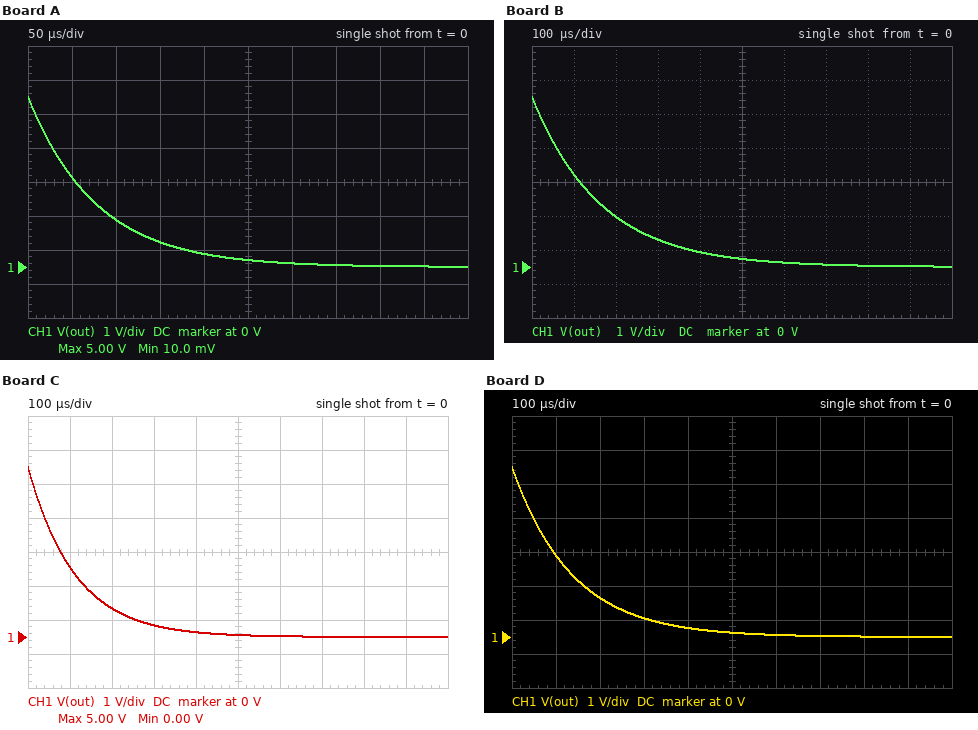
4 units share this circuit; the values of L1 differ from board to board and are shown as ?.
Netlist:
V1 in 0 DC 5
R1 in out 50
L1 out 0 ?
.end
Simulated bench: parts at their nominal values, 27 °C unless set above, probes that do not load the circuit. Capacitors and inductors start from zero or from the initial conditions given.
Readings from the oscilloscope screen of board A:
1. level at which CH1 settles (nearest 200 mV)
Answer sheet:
0 V
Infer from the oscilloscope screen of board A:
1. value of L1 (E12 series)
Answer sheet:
3.9 mH
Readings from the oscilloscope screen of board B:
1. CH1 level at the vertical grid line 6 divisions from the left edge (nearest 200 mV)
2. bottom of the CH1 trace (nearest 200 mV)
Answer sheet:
200 mV
0 V
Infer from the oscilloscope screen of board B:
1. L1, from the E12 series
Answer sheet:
8.2 mH
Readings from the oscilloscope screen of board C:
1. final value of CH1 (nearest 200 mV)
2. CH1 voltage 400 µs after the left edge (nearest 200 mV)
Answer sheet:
0 V
200 mV
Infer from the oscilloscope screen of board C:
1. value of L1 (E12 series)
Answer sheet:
5.6 mH
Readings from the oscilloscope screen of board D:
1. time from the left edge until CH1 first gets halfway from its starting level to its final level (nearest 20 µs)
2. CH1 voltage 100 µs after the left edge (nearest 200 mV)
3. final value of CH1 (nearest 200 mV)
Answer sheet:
100 µs
2.4 V
0 V
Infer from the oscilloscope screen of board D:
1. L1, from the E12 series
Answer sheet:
6.8 mH
